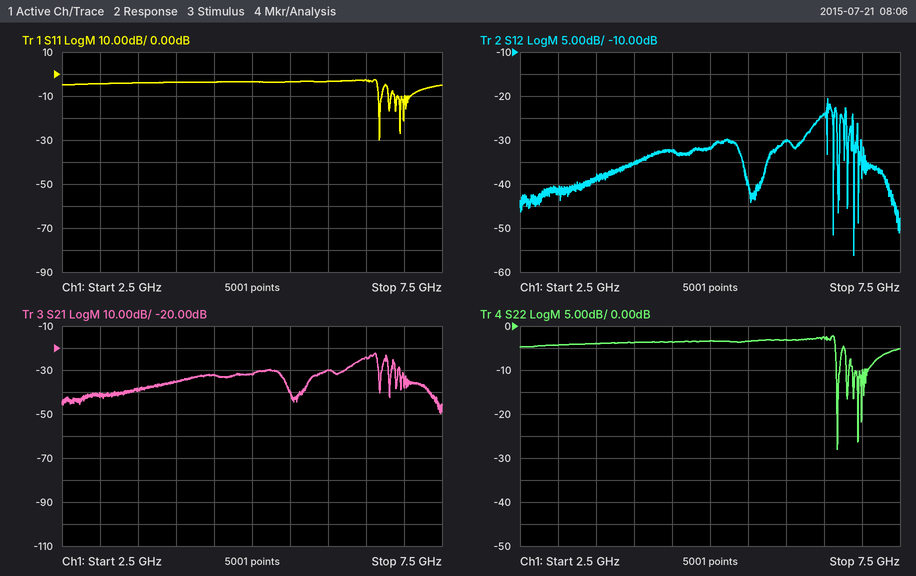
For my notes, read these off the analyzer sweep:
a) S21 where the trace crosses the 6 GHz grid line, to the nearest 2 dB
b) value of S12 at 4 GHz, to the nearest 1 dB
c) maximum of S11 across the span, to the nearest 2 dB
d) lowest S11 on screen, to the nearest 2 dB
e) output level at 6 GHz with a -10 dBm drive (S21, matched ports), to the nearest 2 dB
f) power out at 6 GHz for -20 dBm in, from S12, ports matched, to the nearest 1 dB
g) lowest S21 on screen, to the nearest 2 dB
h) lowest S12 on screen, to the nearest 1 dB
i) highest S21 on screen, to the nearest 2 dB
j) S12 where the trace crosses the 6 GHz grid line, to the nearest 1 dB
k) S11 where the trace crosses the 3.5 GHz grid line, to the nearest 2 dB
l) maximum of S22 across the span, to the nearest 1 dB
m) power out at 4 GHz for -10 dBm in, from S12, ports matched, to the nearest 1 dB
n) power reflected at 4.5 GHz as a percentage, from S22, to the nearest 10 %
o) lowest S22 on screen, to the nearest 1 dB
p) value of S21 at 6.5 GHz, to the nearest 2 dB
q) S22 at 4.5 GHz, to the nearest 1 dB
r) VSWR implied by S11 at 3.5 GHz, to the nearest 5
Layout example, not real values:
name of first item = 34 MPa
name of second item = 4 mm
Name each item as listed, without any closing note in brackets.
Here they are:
S21 where the trace crosses the 6 GHz grid line, to the nearest 2 dB = -30 dB
value of S12 at 4 GHz, to the nearest 1 dB = -35 dB
maximum of S11 across the span, to the nearest 2 dB = -2 dB
lowest S11 on screen, to the nearest 2 dB = -30 dB
output level at 6 GHz with a -10 dBm drive (S21, matched ports), to the nearest 2 dB = -40 dBm
power out at 6 GHz for -20 dBm in, from S12, ports matched, to the nearest 1 dB = -50 dBm
lowest S21 on screen, to the nearest 2 dB = -50 dB
lowest S12 on screen, to the nearest 1 dB = -56 dB
highest S21 on screen, to the nearest 2 dB = -22 dB
S12 where the trace crosses the 6 GHz grid line, to the nearest 1 dB = -30 dB
S11 where the trace crosses the 3.5 GHz grid line, to the nearest 2 dB = -4 dB
maximum of S22 across the span, to the nearest 1 dB = -2 dB
power out at 4 GHz for -10 dBm in, from S12, ports matched, to the nearest 1 dB = -45 dBm
power reflected at 4.5 GHz as a percentage, from S22, to the nearest 10 % = 40 %
lowest S22 on screen, to the nearest 1 dB = -28 dB
value of S21 at 6.5 GHz, to the nearest 2 dB = -24 dB
S22 at 4.5 GHz, to the nearest 1 dB = -4 dB
VSWR implied by S11 at 3.5 GHz, to the nearest 5 = 5
